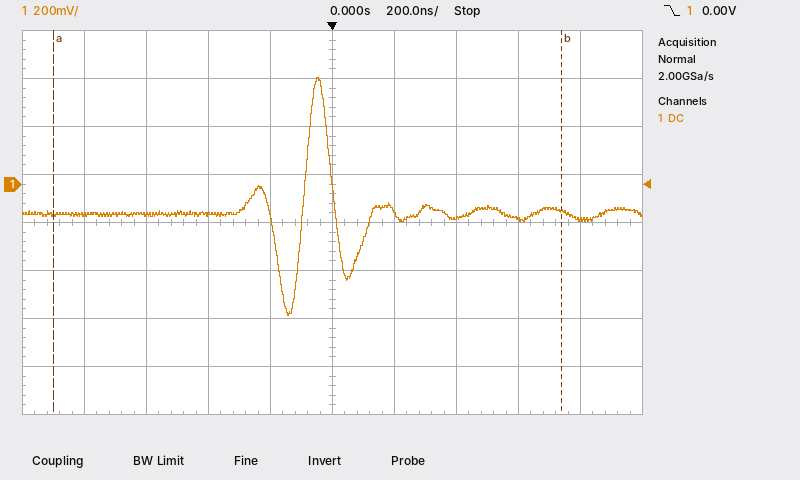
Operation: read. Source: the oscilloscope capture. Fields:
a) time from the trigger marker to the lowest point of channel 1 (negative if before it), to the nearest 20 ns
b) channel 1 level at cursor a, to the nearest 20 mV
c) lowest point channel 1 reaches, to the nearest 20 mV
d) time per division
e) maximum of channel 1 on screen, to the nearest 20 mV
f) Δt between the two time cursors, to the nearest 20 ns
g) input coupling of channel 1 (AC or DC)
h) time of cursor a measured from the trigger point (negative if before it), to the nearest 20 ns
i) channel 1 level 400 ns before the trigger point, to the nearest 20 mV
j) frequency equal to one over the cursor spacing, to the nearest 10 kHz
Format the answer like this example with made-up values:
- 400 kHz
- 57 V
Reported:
- -140 ns
- -120 mV
- -540 mV
- 200 ns
- 440 mV
- 1.64 µs
- DC
- -900 ns
- -120 mV
- 610 kHz
